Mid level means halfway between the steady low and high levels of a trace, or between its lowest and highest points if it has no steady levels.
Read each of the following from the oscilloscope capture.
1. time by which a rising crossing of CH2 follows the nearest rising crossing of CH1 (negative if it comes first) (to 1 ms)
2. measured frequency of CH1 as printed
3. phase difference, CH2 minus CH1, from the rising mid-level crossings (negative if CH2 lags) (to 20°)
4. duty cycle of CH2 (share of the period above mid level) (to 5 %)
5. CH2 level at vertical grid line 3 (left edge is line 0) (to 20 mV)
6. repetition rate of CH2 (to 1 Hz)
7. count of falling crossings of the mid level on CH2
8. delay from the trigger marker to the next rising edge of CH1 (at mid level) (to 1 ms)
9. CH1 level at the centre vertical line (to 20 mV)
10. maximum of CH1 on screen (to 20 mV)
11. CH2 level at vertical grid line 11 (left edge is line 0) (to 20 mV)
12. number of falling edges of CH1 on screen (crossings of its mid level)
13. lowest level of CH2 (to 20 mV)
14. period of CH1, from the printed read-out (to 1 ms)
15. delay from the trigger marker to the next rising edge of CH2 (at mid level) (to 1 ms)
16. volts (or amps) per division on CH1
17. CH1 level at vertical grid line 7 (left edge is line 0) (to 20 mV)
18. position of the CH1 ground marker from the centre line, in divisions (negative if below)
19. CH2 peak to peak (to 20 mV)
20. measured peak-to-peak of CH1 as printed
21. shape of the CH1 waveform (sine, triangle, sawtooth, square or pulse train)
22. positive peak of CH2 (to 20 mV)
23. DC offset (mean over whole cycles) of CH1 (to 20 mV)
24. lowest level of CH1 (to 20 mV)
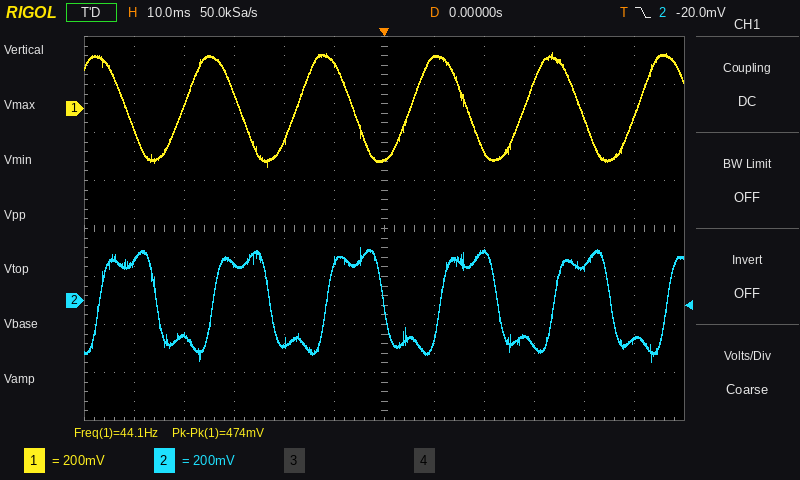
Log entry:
+6 ms
44.1 Hz
-100°
50 %
160 mV
44 Hz
5
5 ms
-220 mV
240 mV
-160 mV
5
-260 mV
23 ms
11 ms
200 mV
220 mV
+2.5 div
480 mV
474 mV
sine
220 mV
0 mV
-240 mV
